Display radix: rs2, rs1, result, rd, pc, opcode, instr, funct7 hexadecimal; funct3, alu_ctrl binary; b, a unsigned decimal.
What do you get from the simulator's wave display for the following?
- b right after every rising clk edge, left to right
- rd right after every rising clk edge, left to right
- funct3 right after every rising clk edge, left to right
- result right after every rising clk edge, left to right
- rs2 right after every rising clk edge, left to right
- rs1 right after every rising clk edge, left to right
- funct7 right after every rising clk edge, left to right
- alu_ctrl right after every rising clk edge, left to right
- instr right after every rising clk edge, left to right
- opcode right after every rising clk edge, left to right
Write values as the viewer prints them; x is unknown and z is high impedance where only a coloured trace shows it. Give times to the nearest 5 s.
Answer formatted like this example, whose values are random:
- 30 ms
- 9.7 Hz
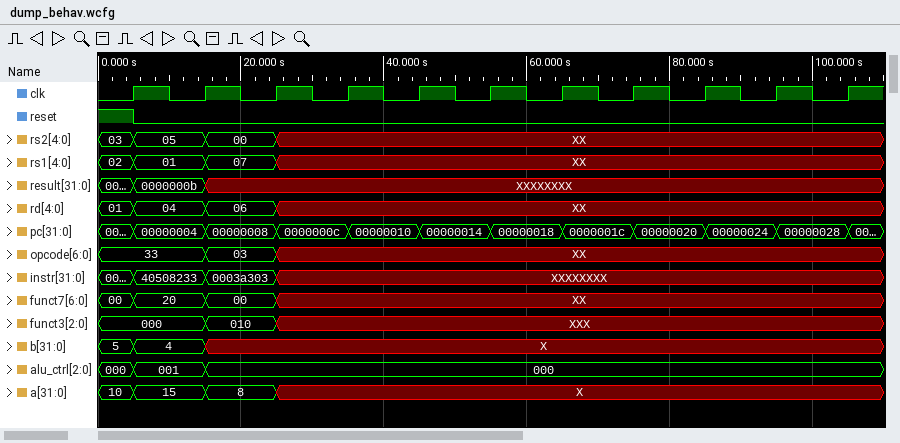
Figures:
- 4, X, X, X, X, X, X, X, X, X, X
- 04, 06, XX, XX, XX, XX, XX, XX, XX, XX, XX
- 000, 010, XXX, XXX, XXX, XXX, XXX, XXX, XXX, XXX, XXX
- 0000000b, XXXXXXXX, XXXXXXXX, XXXXXXXX, XXXXXXXX, XXXXXXXX, XXXXXXXX, XXXXXXXX, XXXXXXXX, XXXXXXXX, XXXXXXXX
- 05, 00, XX, XX, XX, XX, XX, XX, XX, XX, XX
- 01, 07, XX, XX, XX, XX, XX, XX, XX, XX, XX
- 20, 00, XX, XX, XX, XX, XX, XX, XX, XX, XX
- 001, 000, 000, 000, 000, 000, 000, 000, 000, 000, 000
- 40508233, 0003a303, XXXXXXXX, XXXXXXXX, XXXXXXXX, XXXXXXXX, XXXXXXXX, XXXXXXXX, XXXXXXXX, XXXXXXXX, XXXXXXXX
- 33, 03, XX, XX, XX, XX, XX, XX, XX, XX, XX
